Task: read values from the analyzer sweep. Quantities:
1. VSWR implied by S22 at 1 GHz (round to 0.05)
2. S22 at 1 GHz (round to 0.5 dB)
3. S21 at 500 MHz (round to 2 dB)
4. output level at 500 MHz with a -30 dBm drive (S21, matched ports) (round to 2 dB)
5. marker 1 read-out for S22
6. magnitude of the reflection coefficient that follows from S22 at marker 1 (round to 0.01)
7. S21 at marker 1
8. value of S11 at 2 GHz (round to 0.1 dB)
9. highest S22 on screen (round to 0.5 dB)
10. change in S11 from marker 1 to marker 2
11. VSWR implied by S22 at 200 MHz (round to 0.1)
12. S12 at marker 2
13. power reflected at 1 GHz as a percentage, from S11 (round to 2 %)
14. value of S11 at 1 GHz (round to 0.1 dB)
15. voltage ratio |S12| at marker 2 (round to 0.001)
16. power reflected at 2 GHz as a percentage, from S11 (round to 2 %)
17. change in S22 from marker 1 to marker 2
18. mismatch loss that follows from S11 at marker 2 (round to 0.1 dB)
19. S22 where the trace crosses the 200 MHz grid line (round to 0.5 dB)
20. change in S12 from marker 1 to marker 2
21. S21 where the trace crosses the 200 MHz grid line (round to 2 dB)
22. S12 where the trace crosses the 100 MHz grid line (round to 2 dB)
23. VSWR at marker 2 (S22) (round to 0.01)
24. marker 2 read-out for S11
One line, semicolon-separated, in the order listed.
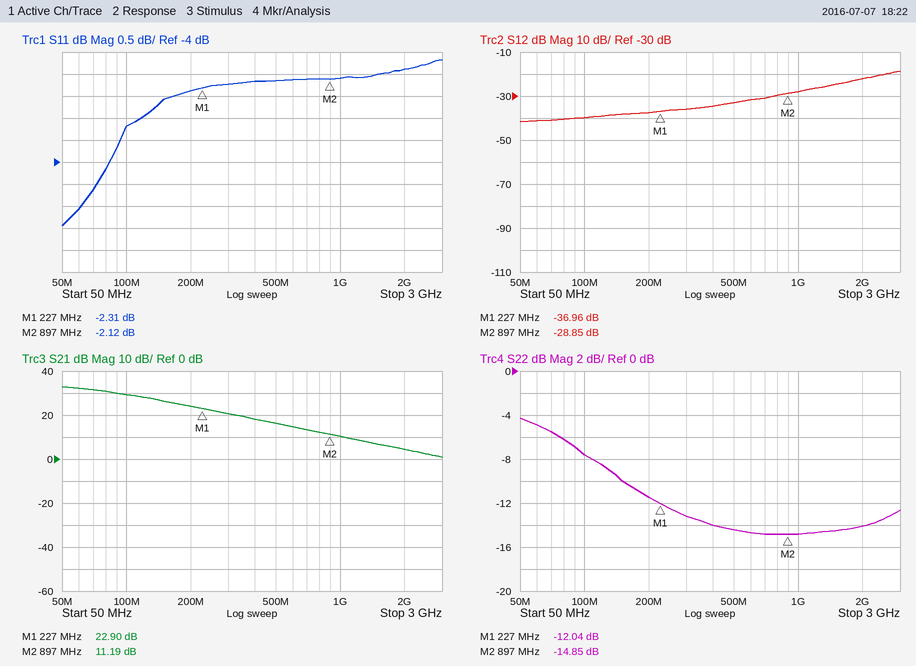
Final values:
1.45; -15.0 dB; 16 dB; -14 dBm; -12.04 dB; 0.25; 22.90 dB; -1.9 dB; -4.5 dB; 0.19 dB; 1.7; -28.85 dB; 62 %; -2.1 dB; 0.036; 64 %; -2.81 dB; 4.1 dB; -11.5 dB; 8.11 dB; 24 dB; -40 dB; 1.44; -2.12 dB
